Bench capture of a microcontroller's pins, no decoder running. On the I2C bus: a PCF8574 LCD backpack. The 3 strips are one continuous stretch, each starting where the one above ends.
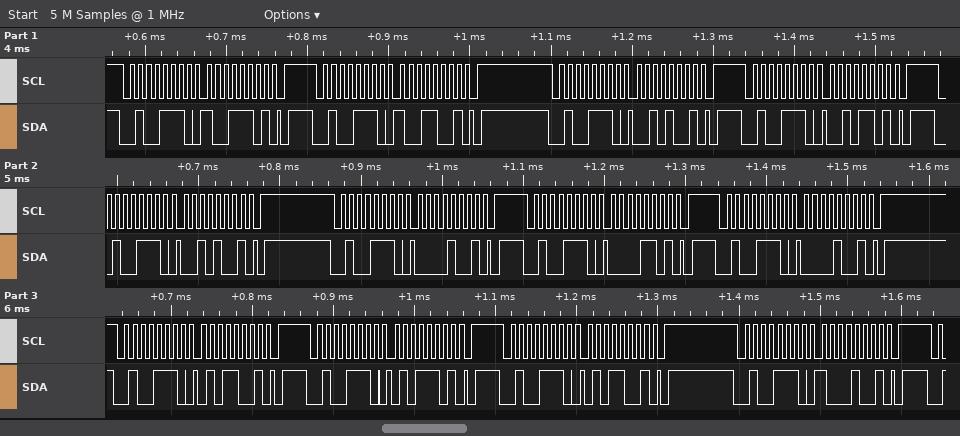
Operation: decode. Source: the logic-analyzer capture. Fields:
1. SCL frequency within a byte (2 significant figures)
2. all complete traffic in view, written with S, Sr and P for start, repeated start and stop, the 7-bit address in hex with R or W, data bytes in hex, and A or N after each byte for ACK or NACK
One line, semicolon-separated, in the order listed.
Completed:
100 kHz; S 27W A 9D A P S 27W A 99 A P S 27W A 29 A P S 27W A 2D A P S 27W A 29 A P S 27W A 09 A P S 27W A 0D A P S 27W A 09 A P S 27W A 59 A P S 27W A 5D A P S 27W A 59 A P S 27W A 89 A P
